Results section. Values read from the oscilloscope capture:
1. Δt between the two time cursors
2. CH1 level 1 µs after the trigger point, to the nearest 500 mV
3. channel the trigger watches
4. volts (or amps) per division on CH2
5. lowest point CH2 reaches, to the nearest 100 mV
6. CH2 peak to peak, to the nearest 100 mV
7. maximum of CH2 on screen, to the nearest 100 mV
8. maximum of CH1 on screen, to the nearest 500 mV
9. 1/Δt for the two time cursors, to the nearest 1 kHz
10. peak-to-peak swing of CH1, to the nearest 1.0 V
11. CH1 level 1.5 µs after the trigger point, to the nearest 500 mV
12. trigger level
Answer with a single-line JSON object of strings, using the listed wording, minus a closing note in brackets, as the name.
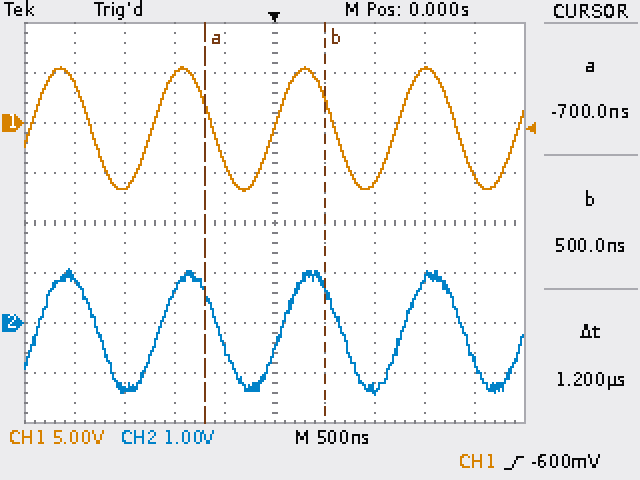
{"Δt between the two time cursors": "1.2 µs", "CH1 level 1 µs after the trigger point, to the nearest 500 mV": "-6.0 V", "channel the trigger watches": "CH1", "volts (or amps) per division on CH2": "1 V", "lowest point CH2 reaches, to the nearest 100 mV": "-1.4 V", "CH2 peak to peak, to the nearest 100 mV": "2.5 V", "maximum of CH2 on screen, to the nearest 100 mV": "1.1 V", "maximum of CH1 on screen, to the nearest 500 mV": "5.5 V", "1/Δt for the two time cursors, to the nearest 1 kHz": "833 kHz", "peak-to-peak swing of CH1, to the nearest 1.0 V": "12.0 V", "CH1 level 1.5 µs after the trigger point, to the nearest 500 mV": "5.5 V", "trigger level": "-600 mV"}
